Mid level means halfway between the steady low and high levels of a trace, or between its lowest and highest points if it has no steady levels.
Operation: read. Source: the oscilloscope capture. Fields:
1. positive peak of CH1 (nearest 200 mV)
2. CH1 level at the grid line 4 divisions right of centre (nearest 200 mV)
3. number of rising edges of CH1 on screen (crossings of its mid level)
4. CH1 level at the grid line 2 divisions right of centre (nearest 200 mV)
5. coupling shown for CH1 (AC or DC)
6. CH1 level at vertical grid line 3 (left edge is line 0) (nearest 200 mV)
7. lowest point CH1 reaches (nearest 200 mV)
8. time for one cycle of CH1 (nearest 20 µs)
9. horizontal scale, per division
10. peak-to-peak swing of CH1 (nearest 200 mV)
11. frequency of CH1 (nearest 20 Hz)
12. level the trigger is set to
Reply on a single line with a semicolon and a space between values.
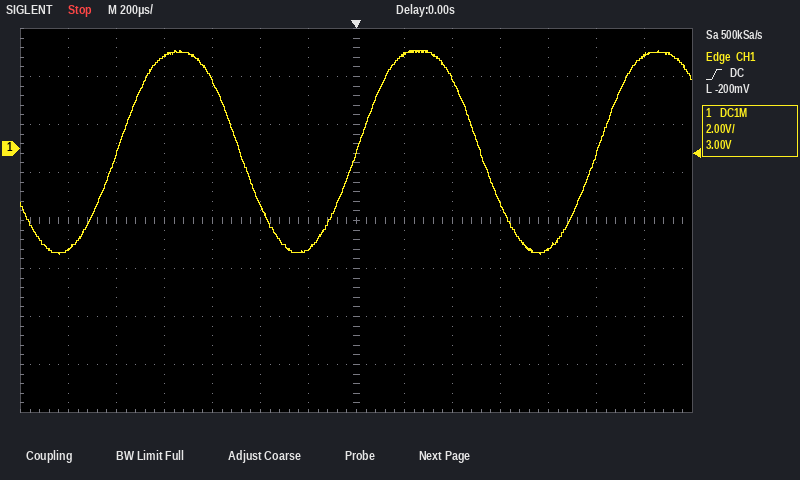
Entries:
4.0 V; -4.2 V; 3; 3.0 V; DC; 3.8 V; -4.4 V; 1.00 ms; 200 µs; 8.4 V; 1.00 kHz; -200 mV
